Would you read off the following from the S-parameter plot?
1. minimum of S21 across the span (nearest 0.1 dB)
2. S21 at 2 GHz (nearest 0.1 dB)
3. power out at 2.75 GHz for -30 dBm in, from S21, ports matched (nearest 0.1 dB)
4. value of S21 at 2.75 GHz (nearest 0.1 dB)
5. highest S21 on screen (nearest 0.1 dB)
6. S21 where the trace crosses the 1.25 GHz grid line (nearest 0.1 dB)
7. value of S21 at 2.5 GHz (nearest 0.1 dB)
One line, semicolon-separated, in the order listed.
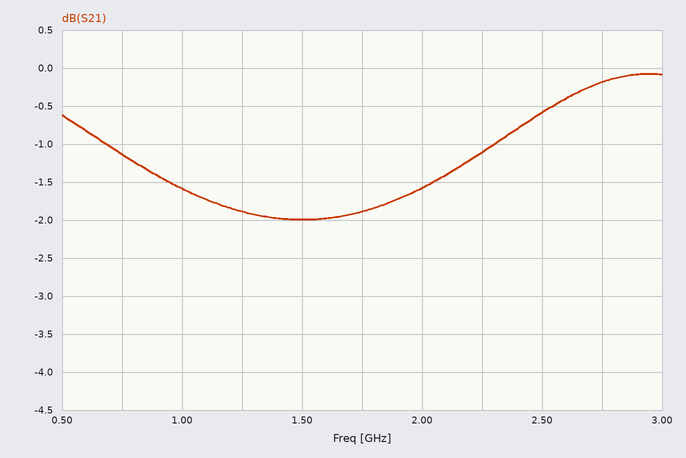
-2.0 dB; -1.6 dB; -30.2 dBm; -0.2 dB; -0.1 dB; -1.9 dB; -0.6 dB
